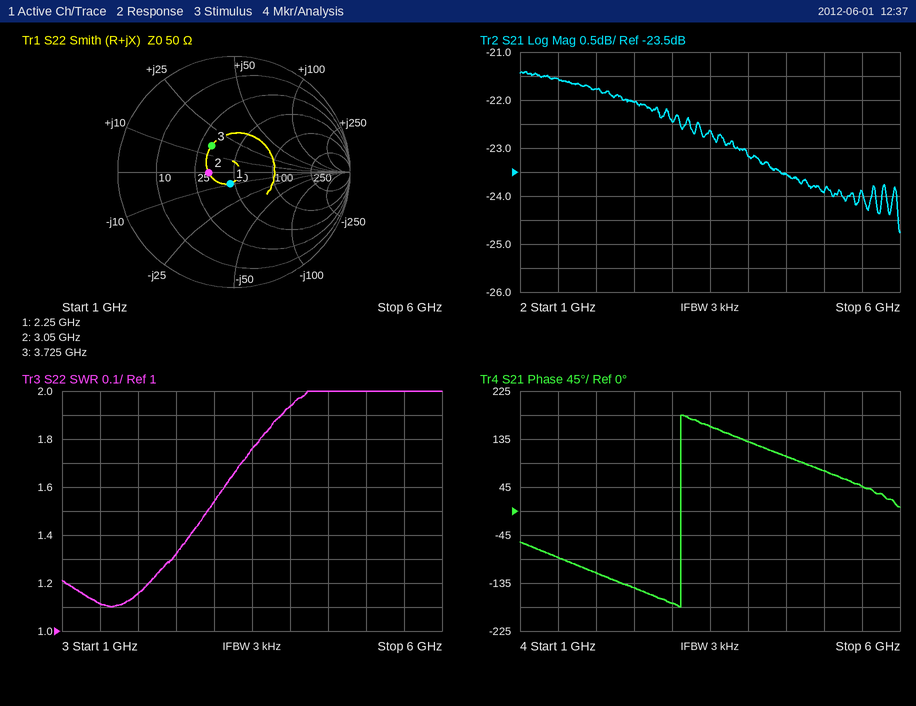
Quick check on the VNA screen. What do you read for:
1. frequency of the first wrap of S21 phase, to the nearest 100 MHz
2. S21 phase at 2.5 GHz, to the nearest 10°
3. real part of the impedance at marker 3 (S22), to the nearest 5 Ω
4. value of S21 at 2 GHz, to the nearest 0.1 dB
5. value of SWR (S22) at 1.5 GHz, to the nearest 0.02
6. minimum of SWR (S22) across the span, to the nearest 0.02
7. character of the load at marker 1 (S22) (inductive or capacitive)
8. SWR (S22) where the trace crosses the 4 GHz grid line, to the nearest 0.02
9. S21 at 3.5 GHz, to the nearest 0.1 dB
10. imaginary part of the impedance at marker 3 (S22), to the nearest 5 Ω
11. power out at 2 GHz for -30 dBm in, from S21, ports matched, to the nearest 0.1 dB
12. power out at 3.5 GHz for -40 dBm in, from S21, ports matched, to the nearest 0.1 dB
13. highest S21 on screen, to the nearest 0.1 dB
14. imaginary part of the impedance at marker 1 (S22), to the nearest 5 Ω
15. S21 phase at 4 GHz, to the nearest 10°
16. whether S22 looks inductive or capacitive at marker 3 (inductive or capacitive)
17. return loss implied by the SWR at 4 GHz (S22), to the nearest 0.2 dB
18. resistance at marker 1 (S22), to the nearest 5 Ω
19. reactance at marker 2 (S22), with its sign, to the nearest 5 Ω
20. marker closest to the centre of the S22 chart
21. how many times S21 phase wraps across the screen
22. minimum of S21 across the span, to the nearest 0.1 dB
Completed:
3.1 GHz
-140°
30 Ω
-21.8 dB
1.12
1.10
capacitive
1.94
-22.6 dB
+15 Ω
-51.8 dBm
-62.6 dBm
-21.4 dB
-10 Ω
130°
inductive
10.0 dB
45 Ω
0 Ω
marker 1
1
-24.8 dB
